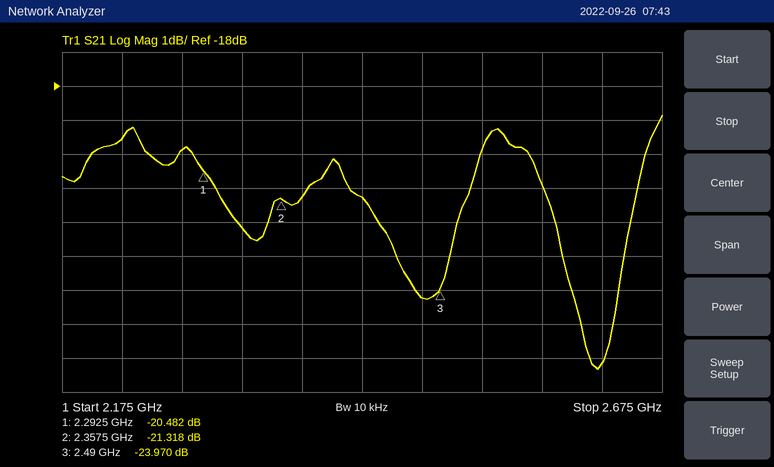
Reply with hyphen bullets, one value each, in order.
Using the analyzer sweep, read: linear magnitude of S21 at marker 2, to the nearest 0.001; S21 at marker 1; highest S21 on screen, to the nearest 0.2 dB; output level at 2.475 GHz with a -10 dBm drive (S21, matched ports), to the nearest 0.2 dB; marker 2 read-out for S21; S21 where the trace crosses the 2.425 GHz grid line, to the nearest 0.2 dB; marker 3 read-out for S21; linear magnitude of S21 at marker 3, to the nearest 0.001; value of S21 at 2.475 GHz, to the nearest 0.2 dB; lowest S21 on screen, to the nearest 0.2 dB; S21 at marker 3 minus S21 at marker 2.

- 0.086
- -20.482 dB
- -18.8 dB
- -34.2 dBm
- -21.318 dB
- -21.2 dB
- -23.970 dB
- 0.063
- -24.2 dB
- -26.4 dB
- -2.652 dB
